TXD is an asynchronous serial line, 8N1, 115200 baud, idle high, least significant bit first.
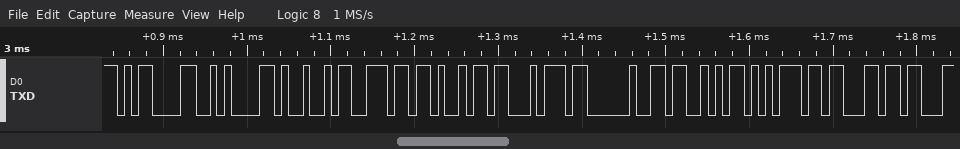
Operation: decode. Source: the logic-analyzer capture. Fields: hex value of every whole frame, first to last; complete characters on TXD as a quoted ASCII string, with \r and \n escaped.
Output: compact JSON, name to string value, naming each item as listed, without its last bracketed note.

{"hex value of every whole frame, first to last": "0x0D 0x0A 0x49 0x6E 0x69 0x74 0x20 0x53 0x75 0x63", "complete characters on TXD as a quoted ASCII string, with \\r and \\n escaped": "\"\\r\\nInit Suc\""}
